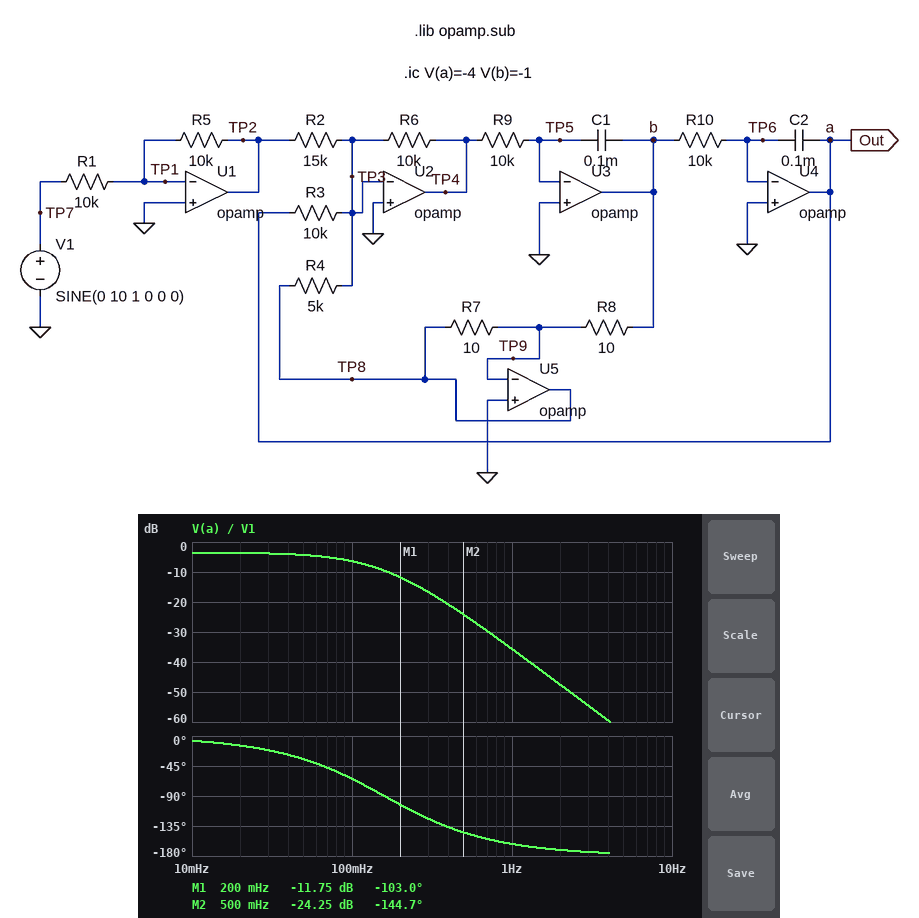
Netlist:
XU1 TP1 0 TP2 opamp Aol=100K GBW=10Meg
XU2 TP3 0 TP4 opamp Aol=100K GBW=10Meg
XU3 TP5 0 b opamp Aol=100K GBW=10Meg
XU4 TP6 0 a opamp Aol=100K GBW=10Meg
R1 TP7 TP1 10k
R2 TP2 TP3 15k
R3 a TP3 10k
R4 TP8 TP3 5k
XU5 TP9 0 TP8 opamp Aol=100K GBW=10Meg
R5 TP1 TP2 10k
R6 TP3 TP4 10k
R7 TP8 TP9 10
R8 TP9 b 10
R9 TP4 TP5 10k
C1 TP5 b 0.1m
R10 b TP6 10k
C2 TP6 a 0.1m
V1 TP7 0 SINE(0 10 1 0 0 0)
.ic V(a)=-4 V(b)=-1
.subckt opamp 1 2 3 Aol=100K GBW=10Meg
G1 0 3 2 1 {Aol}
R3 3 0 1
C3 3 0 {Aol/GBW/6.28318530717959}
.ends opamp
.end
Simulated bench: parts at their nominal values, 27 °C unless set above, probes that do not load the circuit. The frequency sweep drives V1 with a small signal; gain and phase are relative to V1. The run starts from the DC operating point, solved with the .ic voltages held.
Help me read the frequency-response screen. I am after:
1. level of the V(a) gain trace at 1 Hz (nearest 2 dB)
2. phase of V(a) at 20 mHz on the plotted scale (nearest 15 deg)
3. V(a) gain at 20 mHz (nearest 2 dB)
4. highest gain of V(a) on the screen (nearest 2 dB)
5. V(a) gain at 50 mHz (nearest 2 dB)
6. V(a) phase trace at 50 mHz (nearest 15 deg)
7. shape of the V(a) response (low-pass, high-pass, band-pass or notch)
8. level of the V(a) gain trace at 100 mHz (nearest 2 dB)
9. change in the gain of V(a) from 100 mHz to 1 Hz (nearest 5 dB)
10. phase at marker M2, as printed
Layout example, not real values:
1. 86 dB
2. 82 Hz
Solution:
1. -36 dB
2. -15 deg
3. -4 dB
4. -4 dB
5. -4 dB
6. -30 deg
7. low-pass
8. -6 dB
9. -30 dB
10. -144.7 deg
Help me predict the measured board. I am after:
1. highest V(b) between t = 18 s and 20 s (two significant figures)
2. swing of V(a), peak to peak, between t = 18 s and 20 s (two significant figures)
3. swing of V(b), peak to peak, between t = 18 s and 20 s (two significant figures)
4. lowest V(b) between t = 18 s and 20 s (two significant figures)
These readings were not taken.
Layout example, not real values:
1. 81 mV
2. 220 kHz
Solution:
1. 1.0 V
2. 330 mV
3. 2.1 V
4. -1.0 V
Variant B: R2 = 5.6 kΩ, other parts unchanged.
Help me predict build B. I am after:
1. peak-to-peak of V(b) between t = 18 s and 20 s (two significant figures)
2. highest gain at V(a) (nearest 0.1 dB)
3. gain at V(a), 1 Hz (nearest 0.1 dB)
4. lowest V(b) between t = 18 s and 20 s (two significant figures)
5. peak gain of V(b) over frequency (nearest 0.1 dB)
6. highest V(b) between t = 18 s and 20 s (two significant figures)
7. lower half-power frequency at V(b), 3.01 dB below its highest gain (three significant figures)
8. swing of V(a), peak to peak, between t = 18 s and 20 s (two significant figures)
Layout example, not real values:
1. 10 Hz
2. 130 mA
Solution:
1. 5.5 V
2. 5.0 dB
3. -27.1 dB
4. -2.8 V
5. -1.0 dB
6. 2.8 V
7. 65.9 mHz
8. 880 mV
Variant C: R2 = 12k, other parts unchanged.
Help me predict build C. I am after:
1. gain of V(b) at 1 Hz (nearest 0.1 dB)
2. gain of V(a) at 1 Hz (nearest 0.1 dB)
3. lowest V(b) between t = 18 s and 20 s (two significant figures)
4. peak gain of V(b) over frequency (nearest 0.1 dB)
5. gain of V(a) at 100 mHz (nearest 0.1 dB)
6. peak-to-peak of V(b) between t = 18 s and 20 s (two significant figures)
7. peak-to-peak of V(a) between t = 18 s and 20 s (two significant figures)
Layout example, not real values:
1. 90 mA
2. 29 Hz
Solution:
1. -17.8 dB
2. -33.7 dB
3. -1.3 V
4. -7.6 dB
5. -4.5 dB
6. 2.6 V
7. 410 mV
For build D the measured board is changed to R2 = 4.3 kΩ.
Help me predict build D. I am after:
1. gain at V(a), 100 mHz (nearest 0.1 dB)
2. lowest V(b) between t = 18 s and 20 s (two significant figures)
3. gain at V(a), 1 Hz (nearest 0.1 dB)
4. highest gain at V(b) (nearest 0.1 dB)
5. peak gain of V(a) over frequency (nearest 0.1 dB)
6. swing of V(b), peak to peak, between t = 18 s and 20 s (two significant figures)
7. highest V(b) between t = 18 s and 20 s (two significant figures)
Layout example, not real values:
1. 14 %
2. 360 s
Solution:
1. 4.4 dB
2. -3.6 V
3. -24.8 dB
4. 1.3 dB
5. 7.3 dB
6. 7.2 V
7. 3.6 V
